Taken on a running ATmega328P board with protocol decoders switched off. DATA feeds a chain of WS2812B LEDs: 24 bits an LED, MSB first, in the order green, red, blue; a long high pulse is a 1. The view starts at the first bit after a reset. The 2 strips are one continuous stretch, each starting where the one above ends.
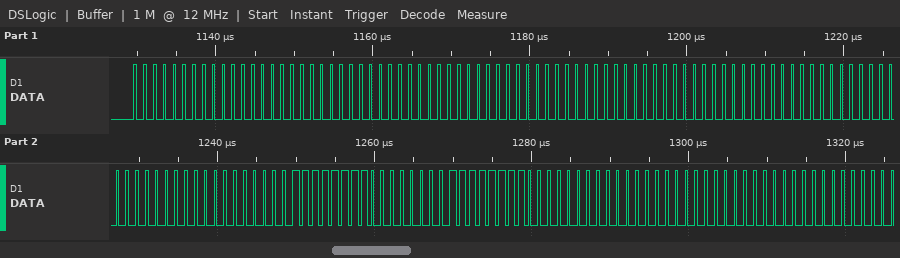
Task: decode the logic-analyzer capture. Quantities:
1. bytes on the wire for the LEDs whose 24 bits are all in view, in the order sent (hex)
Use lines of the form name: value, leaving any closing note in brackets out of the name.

bytes on the wire for the LEDs whose 24 bits are all in view, in the order sent: 00 00 00 00 00 00 00 00 00 00 00 00 FF 00 FF 00 00 00
